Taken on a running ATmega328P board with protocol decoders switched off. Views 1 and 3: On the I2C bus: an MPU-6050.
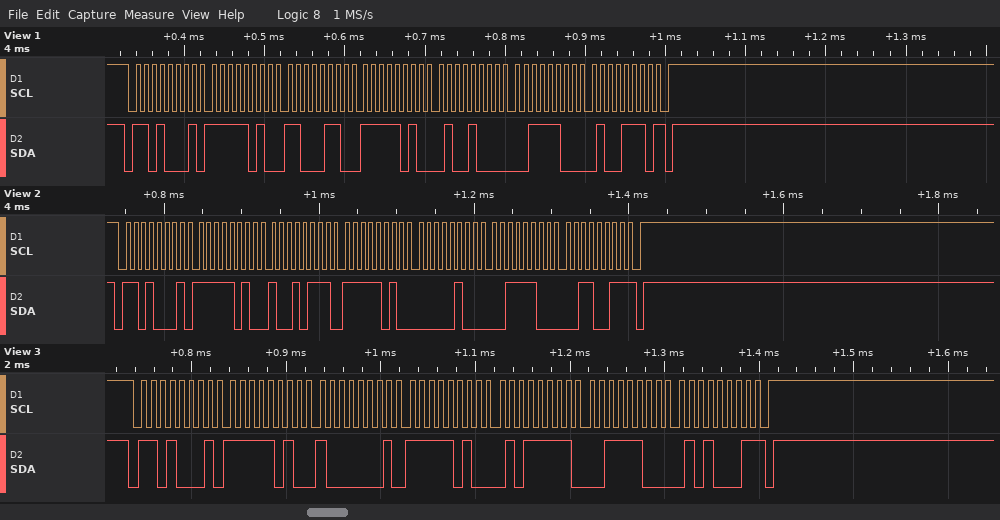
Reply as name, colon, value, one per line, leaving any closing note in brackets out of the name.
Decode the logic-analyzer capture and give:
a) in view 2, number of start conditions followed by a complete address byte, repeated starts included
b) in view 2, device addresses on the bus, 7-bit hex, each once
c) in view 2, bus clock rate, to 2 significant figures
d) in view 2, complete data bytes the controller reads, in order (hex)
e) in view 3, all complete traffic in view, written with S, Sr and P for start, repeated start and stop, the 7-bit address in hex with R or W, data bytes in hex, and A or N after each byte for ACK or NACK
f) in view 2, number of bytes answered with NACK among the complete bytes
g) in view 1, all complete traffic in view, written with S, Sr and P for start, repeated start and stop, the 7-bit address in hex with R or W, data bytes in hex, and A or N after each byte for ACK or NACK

in view 2, number of start conditions followed by a complete address byte, repeated starts included: 1
in view 2, device addresses on the bus, 7-bit hex, each once: 0x68
in view 2, bus clock rate, to 2 significant figures: 100 kHz
in view 2, complete data bytes the controller reads, in order: FA 97 FA 04 3C 33
in view 3, all complete traffic in view, written with S, Sr and P for start, repeated start and stop, the 7-bit address in hex with R or W, data bytes in hex, and A or N after each byte for ACK or NACK: S 68R A FA A 81 A FA A 5F A 3C A 51 N P
in view 2, number of bytes answered with NACK among the complete bytes: 1
in view 1, all complete traffic in view, written with S, Sr and P for start, repeated start and stop, the 7-bit address in hex with R or W, data bytes in hex, and A or N after each byte for ACK or NACK: S 68R A FA A C6 A FA A 48 A 3C A 4E N P
